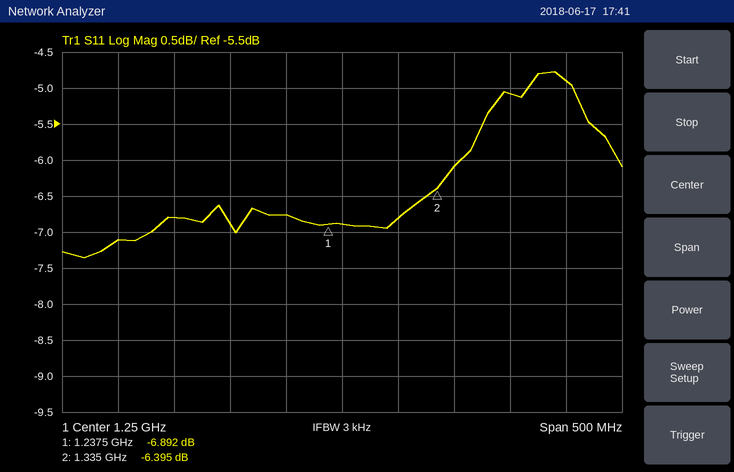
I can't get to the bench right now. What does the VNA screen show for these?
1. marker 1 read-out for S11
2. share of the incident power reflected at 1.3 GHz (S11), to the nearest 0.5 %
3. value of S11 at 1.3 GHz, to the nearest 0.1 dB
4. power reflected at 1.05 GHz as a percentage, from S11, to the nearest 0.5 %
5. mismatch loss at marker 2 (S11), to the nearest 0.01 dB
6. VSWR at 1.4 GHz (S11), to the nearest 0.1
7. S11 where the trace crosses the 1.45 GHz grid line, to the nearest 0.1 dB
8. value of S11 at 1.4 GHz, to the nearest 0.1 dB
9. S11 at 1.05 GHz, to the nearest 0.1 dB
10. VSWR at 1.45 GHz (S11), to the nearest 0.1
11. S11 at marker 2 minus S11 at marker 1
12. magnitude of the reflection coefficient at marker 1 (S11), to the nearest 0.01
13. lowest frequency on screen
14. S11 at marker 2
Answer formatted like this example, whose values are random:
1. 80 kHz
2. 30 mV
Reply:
1. -6.892 dB
2. 21.0 %
3. -6.8 dB
4. 19.5 %
5. 1.13 dB
6. 3.5
7. -4.9 dB
8. -5.1 dB
9. -7.1 dB
10. 3.6
11. 0.497 dB
12. 0.45
13. 1 GHz
14. -6.395 dB
